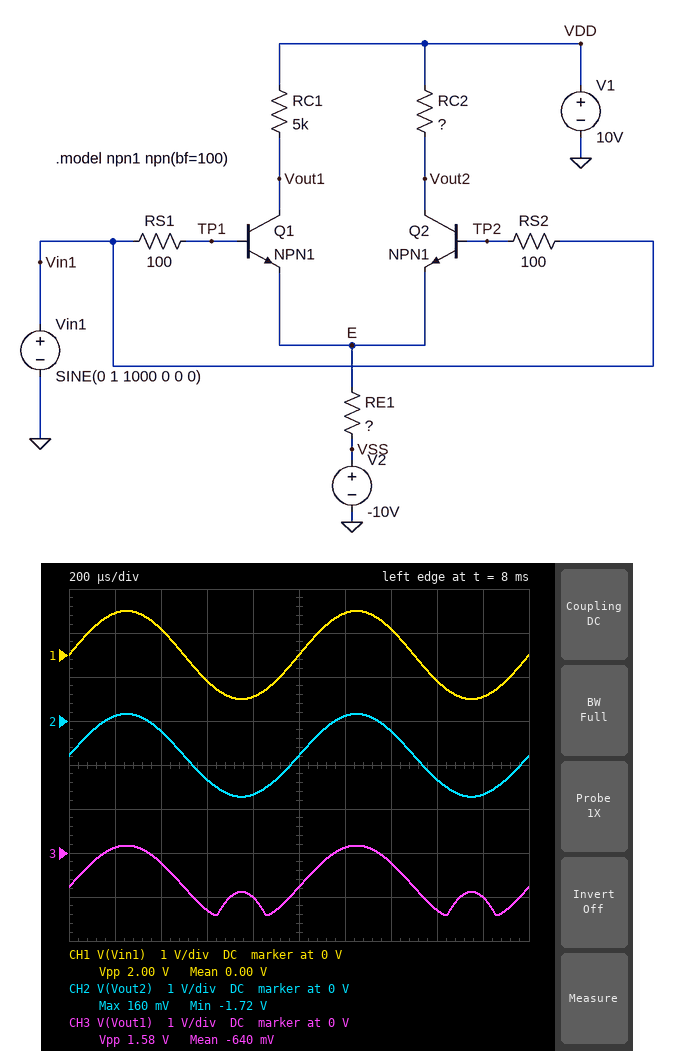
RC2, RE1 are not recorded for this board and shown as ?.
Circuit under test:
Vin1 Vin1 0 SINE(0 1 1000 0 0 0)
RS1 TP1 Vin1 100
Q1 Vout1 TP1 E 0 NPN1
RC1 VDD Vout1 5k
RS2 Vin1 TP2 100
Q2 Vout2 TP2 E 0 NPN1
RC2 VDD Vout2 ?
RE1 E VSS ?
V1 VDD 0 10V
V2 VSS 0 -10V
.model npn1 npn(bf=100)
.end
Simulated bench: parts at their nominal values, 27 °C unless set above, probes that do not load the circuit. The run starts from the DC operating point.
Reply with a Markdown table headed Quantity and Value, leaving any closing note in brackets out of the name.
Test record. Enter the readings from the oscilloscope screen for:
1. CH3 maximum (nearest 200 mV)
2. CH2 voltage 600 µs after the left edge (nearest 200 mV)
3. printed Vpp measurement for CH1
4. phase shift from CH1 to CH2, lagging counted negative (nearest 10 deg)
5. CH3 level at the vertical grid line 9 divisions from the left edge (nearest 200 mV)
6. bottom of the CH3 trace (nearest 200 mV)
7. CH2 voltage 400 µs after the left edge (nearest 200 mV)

| Quantity | Value |
|---|---|
| CH3 maximum | 200 mV |
| CH2 voltage 600 µs after the left edge | -1.4 V |
| printed Vpp measurement for CH1 | 2.00 V |
| phase shift from CH1 to CH2, lagging counted negative | 0 deg |
| CH3 level at the vertical grid line 9 divisions from the left edge | -1.0 V |
| bottom of the CH3 trace | -1.4 V |
| CH2 voltage 400 µs after the left edge | -200 mV |
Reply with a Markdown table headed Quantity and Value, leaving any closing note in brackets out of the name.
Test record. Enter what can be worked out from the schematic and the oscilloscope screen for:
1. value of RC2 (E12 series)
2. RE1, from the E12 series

| Quantity | Value |
|---|---|
| value of RC2 | 8.2 kΩ |
| RE1, from the E12 series | 2.2 kΩ |
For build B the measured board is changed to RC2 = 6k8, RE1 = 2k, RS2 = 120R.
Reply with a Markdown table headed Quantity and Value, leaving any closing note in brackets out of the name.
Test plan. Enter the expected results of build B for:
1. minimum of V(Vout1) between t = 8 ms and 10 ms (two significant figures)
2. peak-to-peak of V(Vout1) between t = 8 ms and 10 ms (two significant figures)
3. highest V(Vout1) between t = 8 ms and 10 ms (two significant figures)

| Quantity | Value |
|---|---|
| minimum of V(Vout1) between t = 8 ms and 10 ms | -1.6 V |
| peak-to-peak of V(Vout1) between t = 8 ms and 10 ms | 1.7 V |
| highest V(Vout1) between t = 8 ms and 10 ms | 140 mV |
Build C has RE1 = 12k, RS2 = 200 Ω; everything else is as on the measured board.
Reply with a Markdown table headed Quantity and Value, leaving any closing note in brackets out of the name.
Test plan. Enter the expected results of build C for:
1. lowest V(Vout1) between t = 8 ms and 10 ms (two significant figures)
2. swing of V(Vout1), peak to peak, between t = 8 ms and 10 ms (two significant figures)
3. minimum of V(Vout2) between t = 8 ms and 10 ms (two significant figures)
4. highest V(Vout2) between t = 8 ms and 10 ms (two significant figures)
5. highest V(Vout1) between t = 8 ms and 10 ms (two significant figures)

| Quantity | Value |
|---|---|
| lowest V(Vout1) between t = 8 ms and 10 ms | 7.9 V |
| swing of V(Vout1), peak to peak, between t = 8 ms and 10 ms | 420 mV |
| minimum of V(Vout2) between t = 8 ms and 10 ms | 6.6 V |
| highest V(Vout2) between t = 8 ms and 10 ms | 7.2 V |
| highest V(Vout1) between t = 8 ms and 10 ms | 8.3 V |
